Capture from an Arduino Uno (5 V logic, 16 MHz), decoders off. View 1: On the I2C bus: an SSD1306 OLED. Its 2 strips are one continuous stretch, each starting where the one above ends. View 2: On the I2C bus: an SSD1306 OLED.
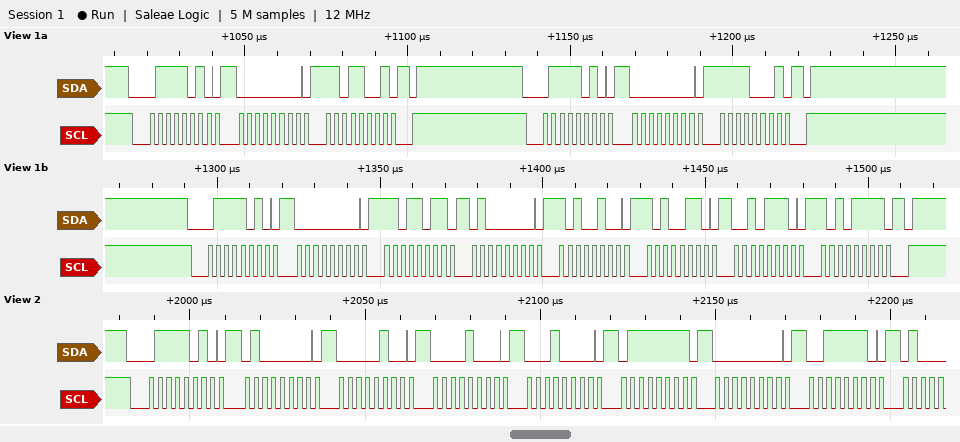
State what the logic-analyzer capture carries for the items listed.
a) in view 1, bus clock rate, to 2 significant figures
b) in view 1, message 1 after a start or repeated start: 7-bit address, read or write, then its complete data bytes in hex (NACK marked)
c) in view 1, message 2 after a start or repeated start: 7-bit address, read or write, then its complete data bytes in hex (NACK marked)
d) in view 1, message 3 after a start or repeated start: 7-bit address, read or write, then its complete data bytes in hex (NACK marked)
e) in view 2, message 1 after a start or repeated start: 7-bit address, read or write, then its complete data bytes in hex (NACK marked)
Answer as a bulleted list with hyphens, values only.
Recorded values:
- 400 kHz
- 0x3D write: 00 D9
- 0x3D write: 00 F1
- 0x3D write: 00 DB 40 A4 A6 2E AF
- 0x3D write: 40 04 08 10 7F 00 3E
